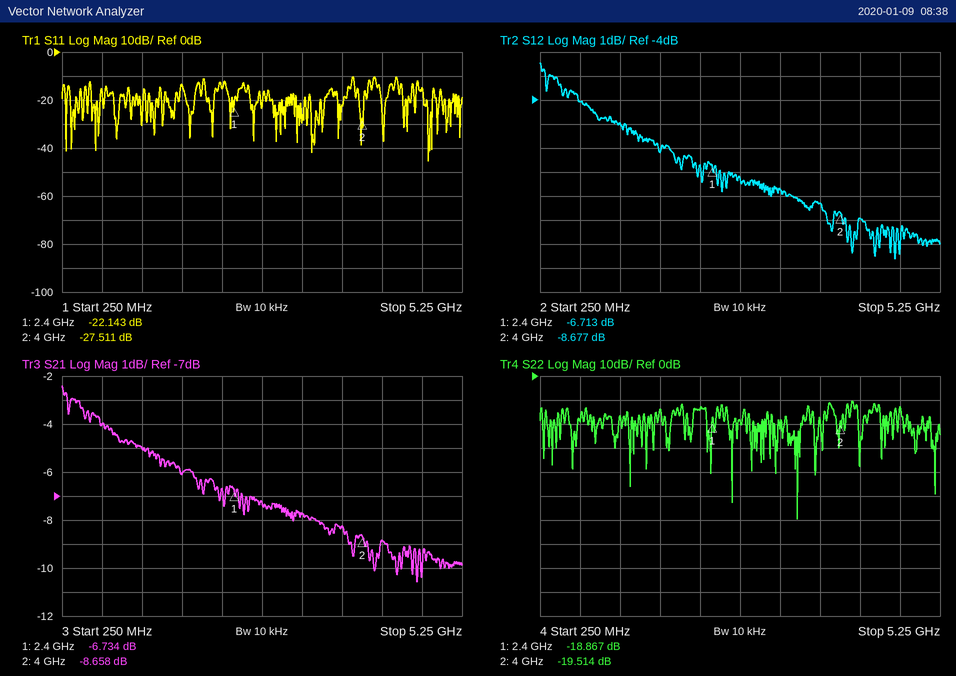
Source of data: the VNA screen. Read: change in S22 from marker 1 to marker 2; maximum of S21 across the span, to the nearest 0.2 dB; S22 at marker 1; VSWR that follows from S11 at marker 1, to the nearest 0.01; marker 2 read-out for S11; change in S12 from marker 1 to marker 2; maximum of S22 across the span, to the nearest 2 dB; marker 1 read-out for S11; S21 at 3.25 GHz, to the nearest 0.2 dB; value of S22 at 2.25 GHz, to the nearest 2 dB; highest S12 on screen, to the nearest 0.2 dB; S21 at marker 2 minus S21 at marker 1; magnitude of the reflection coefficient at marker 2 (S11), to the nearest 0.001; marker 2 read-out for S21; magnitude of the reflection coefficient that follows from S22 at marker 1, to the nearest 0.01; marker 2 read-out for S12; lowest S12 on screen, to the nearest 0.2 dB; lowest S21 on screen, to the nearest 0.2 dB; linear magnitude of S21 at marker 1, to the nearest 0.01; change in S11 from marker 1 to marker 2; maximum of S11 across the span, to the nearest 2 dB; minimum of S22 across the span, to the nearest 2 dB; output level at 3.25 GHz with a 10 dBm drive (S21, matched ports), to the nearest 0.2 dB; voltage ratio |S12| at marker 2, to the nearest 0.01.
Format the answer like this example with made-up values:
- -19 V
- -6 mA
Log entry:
- -0.647 dB
- -2.4 dB
- -18.867 dB
- 1.17
- -27.511 dB
- -1.964 dB
- -10 dB
- -22.143 dB
- -7.8 dB
- -14 dB
- -2.4 dB
- -1.924 dB
- 0.042
- -8.658 dB
- 0.11
- -8.677 dB
- -10.6 dB
- -10.6 dB
- 0.46
- -5.368 dB
- -10 dB
- -60 dB
- 2.2 dBm
- 0.37
